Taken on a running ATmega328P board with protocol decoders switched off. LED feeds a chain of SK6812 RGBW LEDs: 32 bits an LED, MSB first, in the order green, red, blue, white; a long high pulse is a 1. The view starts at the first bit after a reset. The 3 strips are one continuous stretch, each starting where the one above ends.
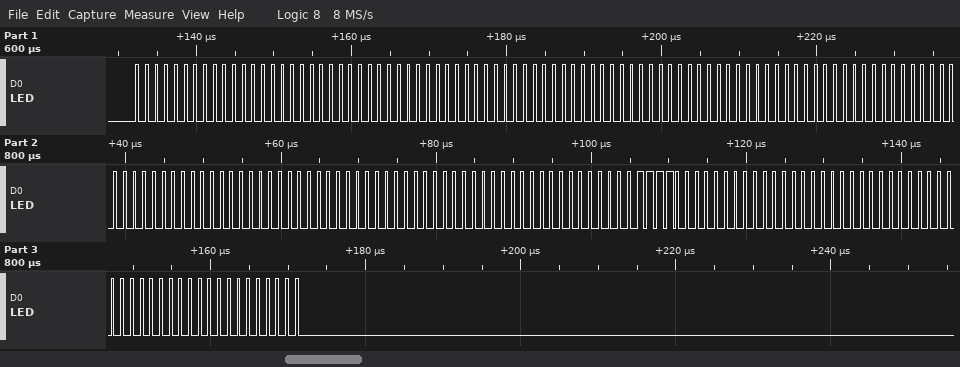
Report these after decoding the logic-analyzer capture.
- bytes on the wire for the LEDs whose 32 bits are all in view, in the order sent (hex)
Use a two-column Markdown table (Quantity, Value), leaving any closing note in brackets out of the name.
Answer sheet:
| Quantity | Value |
|---|---|
| bytes on the wire for the LEDs whose 32 bits are all in view, in the order sent | 00 00 00 00 00 00 00 00 00 00 00 00 00 00 00 00 00 1E 00 00 00 00 00 00 |
